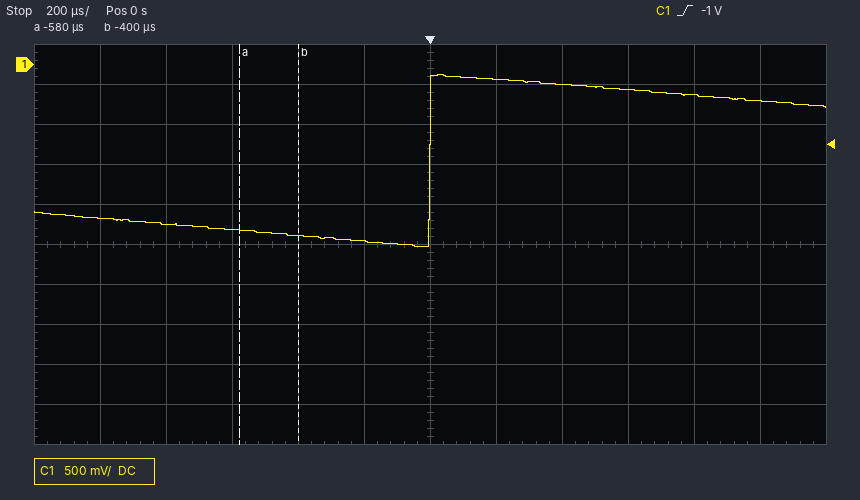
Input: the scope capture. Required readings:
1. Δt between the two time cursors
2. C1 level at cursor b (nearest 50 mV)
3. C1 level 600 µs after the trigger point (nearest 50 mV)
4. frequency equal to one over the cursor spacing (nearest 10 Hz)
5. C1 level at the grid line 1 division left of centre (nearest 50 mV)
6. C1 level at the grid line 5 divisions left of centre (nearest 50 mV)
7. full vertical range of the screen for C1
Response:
180 µs
-2.15 V
-300 mV
5.56 kHz
-2.20 V
-1.90 V
5 V
